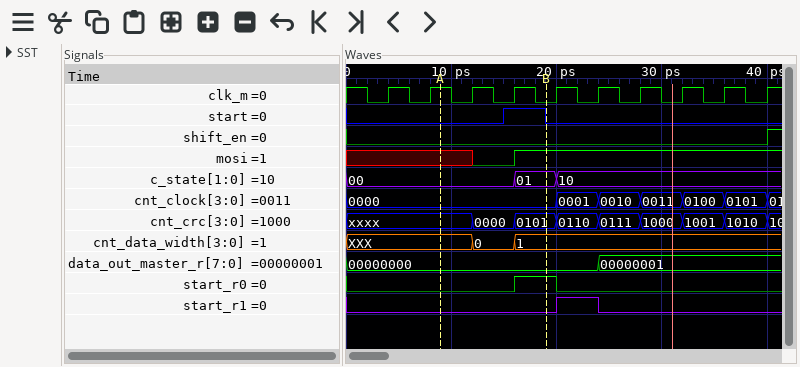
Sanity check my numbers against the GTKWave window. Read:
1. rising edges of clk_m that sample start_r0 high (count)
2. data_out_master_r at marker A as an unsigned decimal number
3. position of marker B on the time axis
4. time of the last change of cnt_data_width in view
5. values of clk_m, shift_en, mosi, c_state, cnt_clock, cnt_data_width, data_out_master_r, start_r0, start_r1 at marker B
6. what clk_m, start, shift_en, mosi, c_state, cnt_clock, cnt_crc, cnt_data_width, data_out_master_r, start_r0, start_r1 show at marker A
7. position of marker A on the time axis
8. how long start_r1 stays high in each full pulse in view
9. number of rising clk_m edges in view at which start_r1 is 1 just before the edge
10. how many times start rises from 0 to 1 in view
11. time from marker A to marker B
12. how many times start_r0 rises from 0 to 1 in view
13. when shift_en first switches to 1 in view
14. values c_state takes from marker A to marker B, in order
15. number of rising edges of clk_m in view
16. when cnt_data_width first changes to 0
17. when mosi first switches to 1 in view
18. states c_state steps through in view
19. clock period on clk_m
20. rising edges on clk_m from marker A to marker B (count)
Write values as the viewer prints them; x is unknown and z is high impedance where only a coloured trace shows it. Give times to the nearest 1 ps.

1
0
19 ps
16 ps
clk_m=0, shift_en=0, mosi=1, c_state=01, cnt_clock=0000, cnt_data_width=1, data_out_master_r=00000000, start_r0=1, start_r1=0
clk_m=1, start=0, shift_en=0, mosi=x, c_state=00, cnt_clock=0000, cnt_crc=xxxx, cnt_data_width=XXX, data_out_master_r=00000000, start_r0=0, start_r1=0
9 ps
4 ps
1
1
10 ps
1
40 ps
00, 01
10
12 ps
16 ps
00, 01, 10
4 ps
2
